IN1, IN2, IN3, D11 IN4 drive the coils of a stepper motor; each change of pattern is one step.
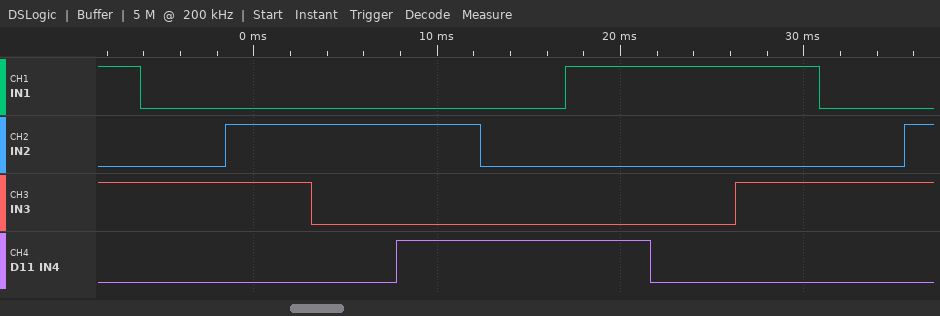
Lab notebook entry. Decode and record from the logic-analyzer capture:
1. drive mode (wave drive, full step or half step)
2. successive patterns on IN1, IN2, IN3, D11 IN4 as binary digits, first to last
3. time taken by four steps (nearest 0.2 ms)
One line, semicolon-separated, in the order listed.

half step; 1010 0010 0110 0100 0101 0001 1001 1000 1010 0010 0110; 18.6 ms
